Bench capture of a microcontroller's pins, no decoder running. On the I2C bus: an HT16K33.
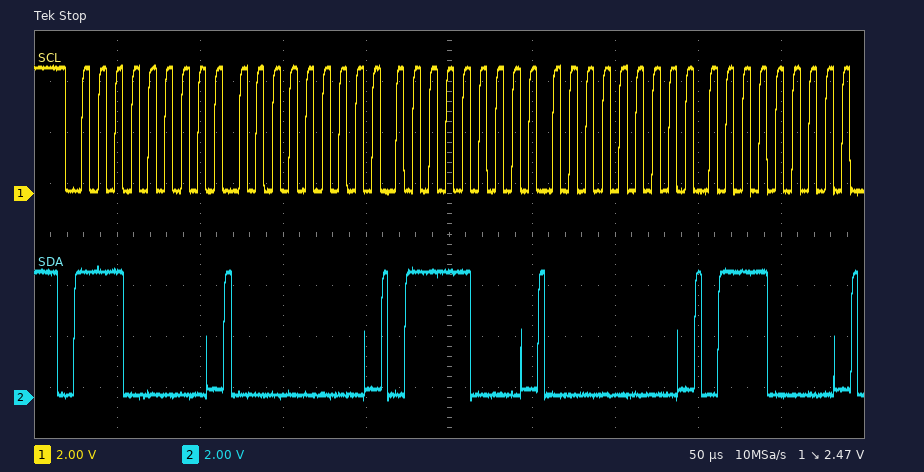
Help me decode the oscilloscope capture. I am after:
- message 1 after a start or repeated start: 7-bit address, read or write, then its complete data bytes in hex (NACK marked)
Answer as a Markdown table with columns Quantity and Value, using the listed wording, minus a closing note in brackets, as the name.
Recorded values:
| Quantity | Value |
|---|---|
| message 1 after a start or repeated start: 7-bit address, read or write, then its complete data bytes in hex | 0x70 write: 00 78 00 70 |
